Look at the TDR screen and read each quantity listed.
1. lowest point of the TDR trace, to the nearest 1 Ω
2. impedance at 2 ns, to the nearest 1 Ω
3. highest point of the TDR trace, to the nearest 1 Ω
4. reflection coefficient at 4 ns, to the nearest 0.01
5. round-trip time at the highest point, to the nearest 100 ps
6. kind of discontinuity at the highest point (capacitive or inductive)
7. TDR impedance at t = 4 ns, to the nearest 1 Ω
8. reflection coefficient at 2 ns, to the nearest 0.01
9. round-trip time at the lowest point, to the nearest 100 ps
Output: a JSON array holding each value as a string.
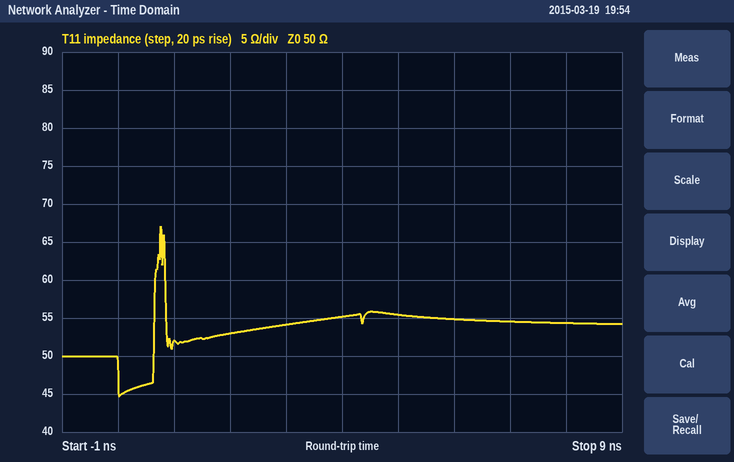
["45 Ω", "53 Ω", "67 Ω", "+0.05", "800 ps", "inductive", "55 Ω", "+0.03", "0.0 ns"]
